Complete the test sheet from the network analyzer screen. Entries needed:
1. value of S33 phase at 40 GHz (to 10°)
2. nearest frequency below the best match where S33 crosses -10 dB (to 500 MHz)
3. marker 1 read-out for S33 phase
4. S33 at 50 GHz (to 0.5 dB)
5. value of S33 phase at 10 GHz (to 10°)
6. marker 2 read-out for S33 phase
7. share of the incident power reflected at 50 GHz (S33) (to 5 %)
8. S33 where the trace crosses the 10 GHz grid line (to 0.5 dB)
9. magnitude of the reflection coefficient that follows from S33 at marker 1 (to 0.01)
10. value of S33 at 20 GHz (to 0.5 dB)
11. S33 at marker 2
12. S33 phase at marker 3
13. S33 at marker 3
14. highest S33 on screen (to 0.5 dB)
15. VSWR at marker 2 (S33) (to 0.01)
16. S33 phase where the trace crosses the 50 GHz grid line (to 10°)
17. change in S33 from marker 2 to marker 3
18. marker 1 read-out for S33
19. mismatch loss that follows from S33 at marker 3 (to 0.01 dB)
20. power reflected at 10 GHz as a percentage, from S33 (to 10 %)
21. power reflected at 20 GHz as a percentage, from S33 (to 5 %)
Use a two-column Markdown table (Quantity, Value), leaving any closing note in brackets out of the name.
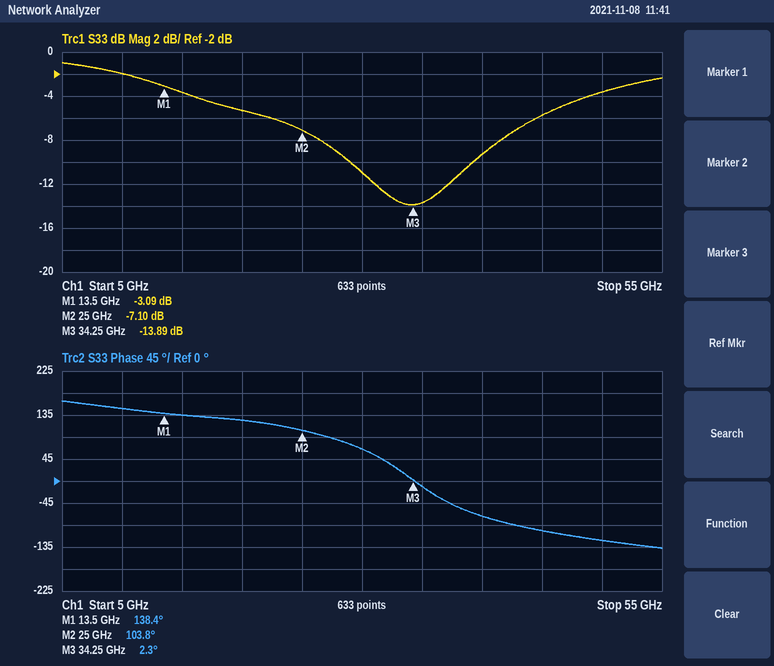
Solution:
| Quantity | Value |
|---|---|
| value of S33 phase at 40 GHz | -70° |
| nearest frequency below the best match where S33 crosses -10 dB | 29.0 GHz |
| marker 1 read-out for S33 phase | 138.4° |
| S33 at 50 GHz | -3.5 dB |
| value of S33 phase at 10 GHz | 150° |
| marker 2 read-out for S33 phase | 103.8° |
| share of the incident power reflected at 50 GHz (S33) | 45 % |
| S33 where the trace crosses the 10 GHz grid line | -2.0 dB |
| magnitude of the reflection coefficient that follows from S33 at marker 1 | 0.70 |
| value of S33 at 20 GHz | -5.5 dB |
| S33 at marker 2 | -7.10 dB |
| S33 phase at marker 3 | 2.3° |
| S33 at marker 3 | -13.89 dB |
| highest S33 on screen | -1.0 dB |
| VSWR at marker 2 (S33) | 2.58 |
| S33 phase where the trace crosses the 50 GHz grid line | -120° |
| change in S33 from marker 2 to marker 3 | -6.79 dB |
| marker 1 read-out for S33 | -3.09 dB |
| mismatch loss that follows from S33 at marker 3 | 0.18 dB |
| power reflected at 10 GHz as a percentage, from S33 | 60 % |
| power reflected at 20 GHz as a percentage, from S33 | 30 % |
